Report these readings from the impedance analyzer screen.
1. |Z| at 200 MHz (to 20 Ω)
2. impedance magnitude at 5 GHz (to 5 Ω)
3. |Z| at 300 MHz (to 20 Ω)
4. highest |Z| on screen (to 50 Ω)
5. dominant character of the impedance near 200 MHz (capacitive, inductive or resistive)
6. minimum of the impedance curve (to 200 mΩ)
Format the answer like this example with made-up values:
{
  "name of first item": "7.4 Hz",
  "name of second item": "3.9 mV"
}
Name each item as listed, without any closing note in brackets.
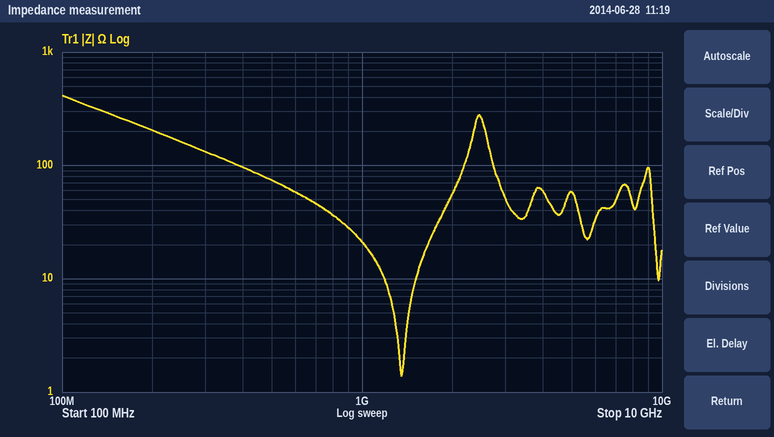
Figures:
{
  "|Z| at 200 MHz": "200 Ω",
  "impedance magnitude at 5 GHz": "60 Ω",
  "|Z| at 300 MHz": "140 Ω",
  "highest |Z| on screen": "400 Ω",
  "dominant character of the impedance near 200 MHz": "capacitive",
  "minimum of the impedance curve": "1.4 Ω"
}
